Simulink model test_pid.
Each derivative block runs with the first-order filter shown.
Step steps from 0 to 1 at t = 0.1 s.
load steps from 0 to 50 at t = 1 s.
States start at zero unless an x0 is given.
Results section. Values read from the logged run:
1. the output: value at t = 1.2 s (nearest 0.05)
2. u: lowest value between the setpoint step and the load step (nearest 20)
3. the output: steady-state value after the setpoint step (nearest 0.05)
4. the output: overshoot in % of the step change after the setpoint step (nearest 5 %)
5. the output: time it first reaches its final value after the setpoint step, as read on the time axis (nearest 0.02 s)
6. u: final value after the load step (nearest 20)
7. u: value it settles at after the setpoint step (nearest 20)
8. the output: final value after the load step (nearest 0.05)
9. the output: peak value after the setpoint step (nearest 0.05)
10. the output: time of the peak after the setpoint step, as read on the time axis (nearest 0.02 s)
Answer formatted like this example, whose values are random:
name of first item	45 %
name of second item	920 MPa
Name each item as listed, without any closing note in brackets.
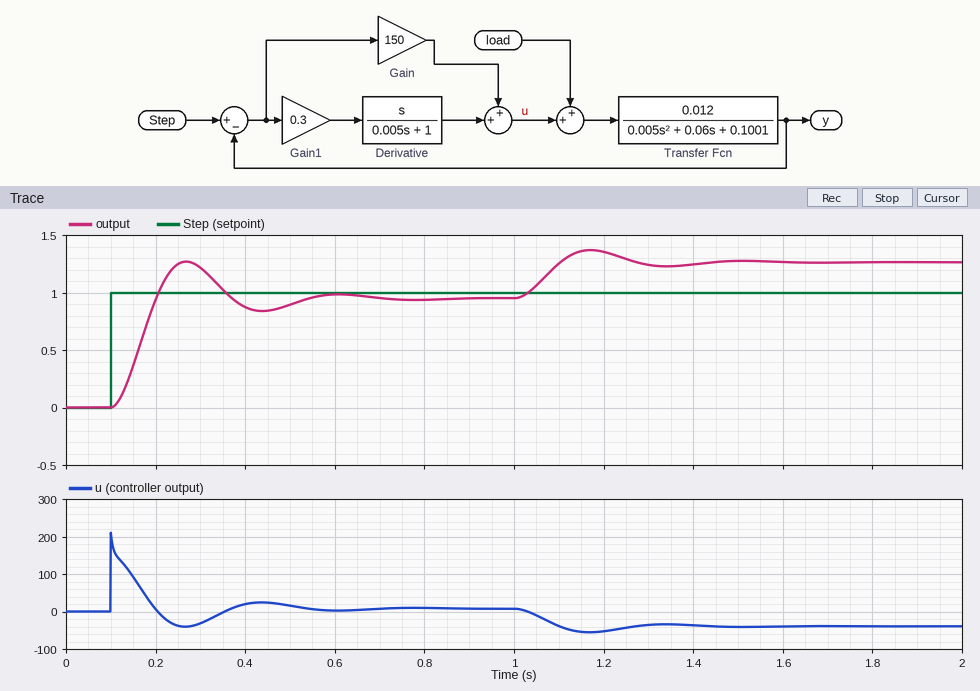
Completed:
the output: value at t = 1.2 s	1.35
u: lowest value between the setpoint step and the load step	-40
the output: steady-state value after the setpoint step	0.95
the output: overshoot in % of the step change after the setpoint step	35 %
the output: time it first reaches its final value after the setpoint step, as read on the time axis	0.20 s
u: final value after the load step	-40
u: value it settles at after the setpoint step	0
the output: final value after the load step	1.25
the output: peak value after the setpoint step	1.25
the output: time of the peak after the setpoint step, as read on the time axis	0.26 s
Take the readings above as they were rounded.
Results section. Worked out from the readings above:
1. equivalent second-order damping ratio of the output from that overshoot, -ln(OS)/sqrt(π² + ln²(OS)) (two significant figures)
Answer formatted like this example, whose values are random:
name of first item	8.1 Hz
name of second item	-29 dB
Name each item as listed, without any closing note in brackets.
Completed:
equivalent second-order damping ratio of the output from that overshoot, -ln(OS)/sqrt(π² + ln²(OS))	0.32
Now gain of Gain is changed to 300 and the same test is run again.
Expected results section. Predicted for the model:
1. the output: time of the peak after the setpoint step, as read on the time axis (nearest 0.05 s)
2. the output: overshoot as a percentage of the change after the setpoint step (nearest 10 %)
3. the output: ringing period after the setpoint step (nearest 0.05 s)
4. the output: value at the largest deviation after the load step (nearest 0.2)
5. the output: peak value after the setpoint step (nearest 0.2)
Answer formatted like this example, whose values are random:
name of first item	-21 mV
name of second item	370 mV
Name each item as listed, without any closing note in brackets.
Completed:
the output: time of the peak after the setpoint step, as read on the time axis	0.20 s
the output: overshoot as a percentage of the change after the setpoint step	50 %
the output: ringing period after the setpoint step	0.25 s
the output: value at the largest deviation after the load step	1.2
the output: peak value after the setpoint step	1.4
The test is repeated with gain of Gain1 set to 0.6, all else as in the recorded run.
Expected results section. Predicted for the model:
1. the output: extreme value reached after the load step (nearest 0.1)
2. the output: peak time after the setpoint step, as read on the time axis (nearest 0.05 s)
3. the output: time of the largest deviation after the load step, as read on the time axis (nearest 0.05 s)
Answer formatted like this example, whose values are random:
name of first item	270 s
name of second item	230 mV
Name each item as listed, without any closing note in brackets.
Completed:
the output: extreme value reached after the load step	1.4
the output: peak time after the setpoint step, as read on the time axis	0.25 s
the output: time of the largest deviation after the load step, as read on the time axis	1.15 s
